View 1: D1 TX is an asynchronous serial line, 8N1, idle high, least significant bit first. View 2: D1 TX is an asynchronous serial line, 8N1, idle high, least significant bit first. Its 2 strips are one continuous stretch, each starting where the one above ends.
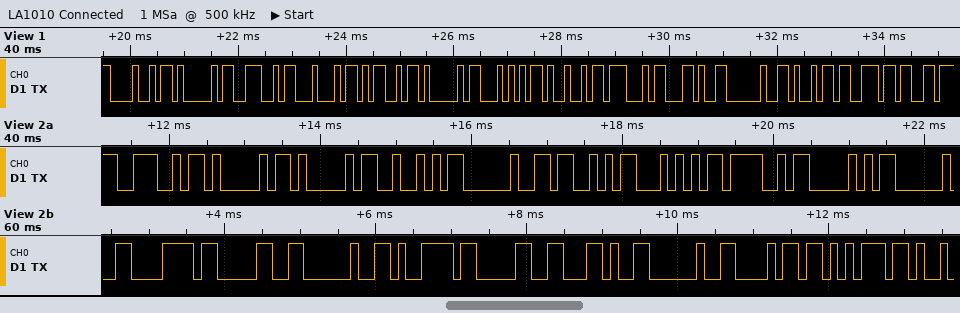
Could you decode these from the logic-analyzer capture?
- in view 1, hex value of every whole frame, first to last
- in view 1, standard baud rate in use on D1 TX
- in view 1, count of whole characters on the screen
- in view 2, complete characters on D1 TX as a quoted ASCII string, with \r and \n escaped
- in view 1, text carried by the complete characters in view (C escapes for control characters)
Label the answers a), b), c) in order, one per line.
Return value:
a) 48 41 4E 44 4D 41 54 49 47 2C 20 69 6E
b) 9600 baud
c) 13
d) "NAAR STOP x0 y0, hu"
e) "HANDMATIG, in"
